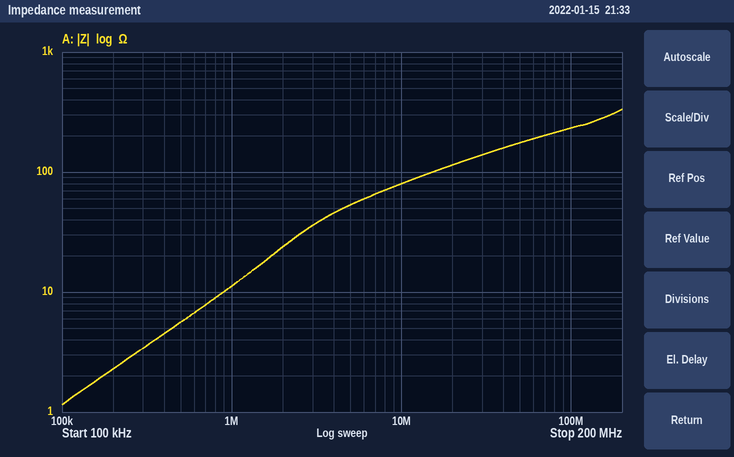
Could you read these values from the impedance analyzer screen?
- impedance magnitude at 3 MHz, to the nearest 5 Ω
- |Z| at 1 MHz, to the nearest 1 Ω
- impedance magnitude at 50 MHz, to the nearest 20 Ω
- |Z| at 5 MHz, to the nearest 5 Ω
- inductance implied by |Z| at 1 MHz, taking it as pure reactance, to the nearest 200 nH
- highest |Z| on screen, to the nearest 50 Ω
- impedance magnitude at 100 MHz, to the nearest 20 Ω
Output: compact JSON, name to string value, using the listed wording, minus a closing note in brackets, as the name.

{"impedance magnitude at 3 MHz, to the nearest 5 Ω": "35 Ω", "|Z| at 1 MHz, to the nearest 1 Ω": "11 Ω", "impedance magnitude at 50 MHz, to the nearest 20 Ω": "180 Ω", "|Z| at 5 MHz, to the nearest 5 Ω": "55 Ω", "inductance implied by |Z| at 1 MHz, taking it as pure reactance, to the nearest 200 nH": "1.8 µH", "highest |Z| on screen, to the nearest 50 Ω": "350 Ω", "impedance magnitude at 100 MHz, to the nearest 20 Ω": "240 Ω"}
